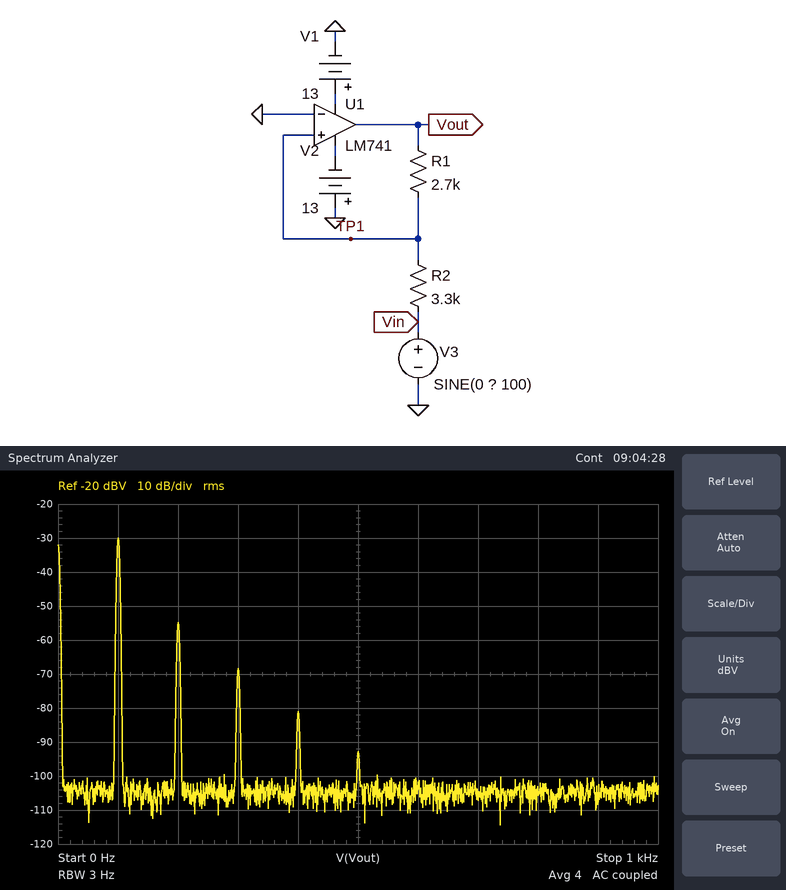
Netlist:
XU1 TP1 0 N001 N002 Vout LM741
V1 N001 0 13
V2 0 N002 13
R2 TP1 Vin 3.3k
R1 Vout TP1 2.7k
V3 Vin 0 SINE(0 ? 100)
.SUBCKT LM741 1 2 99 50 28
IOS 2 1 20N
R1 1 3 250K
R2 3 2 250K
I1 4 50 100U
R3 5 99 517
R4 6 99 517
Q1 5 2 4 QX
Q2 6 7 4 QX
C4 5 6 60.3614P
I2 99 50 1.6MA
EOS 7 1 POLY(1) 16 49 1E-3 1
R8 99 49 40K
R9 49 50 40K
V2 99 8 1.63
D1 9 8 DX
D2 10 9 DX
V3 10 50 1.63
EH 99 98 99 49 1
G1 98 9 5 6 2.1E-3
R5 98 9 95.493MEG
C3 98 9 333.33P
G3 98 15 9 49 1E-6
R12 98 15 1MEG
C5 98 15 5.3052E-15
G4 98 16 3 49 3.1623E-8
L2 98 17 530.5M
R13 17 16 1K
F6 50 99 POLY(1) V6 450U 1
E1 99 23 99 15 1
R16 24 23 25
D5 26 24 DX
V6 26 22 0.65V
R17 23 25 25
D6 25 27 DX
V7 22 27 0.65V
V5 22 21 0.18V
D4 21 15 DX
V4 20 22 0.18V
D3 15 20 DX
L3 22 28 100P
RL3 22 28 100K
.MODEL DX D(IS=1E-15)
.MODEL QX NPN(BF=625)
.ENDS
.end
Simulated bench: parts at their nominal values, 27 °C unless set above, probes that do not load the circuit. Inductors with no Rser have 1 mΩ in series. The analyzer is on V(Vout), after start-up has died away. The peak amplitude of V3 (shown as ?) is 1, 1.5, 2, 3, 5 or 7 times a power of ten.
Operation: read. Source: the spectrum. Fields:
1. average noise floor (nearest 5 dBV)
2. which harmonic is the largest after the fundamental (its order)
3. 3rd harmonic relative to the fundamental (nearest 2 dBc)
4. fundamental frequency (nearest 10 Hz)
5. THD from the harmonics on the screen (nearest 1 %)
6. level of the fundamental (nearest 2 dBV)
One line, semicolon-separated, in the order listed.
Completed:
-105 dBV; 2; -38 dBc; 100 Hz; 6 %; -30 dBV
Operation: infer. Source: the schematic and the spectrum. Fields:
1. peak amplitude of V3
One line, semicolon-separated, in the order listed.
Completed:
7 V
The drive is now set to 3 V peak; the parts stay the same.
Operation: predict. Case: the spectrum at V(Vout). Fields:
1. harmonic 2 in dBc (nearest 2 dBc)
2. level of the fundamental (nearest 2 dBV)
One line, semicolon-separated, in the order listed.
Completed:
-34 dBc; -38 dBV
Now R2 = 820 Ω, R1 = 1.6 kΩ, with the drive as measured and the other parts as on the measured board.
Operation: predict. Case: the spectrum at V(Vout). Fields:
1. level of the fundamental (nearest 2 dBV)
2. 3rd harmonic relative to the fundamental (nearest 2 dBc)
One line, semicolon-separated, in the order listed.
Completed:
20 dBV; -10 dBc
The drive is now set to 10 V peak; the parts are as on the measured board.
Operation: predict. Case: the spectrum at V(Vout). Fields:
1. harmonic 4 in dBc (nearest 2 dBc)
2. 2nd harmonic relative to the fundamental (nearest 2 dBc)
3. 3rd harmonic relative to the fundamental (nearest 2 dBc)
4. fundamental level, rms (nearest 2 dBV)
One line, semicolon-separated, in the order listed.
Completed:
-38 dBc; -20 dBc; -30 dBc; -26 dBV
